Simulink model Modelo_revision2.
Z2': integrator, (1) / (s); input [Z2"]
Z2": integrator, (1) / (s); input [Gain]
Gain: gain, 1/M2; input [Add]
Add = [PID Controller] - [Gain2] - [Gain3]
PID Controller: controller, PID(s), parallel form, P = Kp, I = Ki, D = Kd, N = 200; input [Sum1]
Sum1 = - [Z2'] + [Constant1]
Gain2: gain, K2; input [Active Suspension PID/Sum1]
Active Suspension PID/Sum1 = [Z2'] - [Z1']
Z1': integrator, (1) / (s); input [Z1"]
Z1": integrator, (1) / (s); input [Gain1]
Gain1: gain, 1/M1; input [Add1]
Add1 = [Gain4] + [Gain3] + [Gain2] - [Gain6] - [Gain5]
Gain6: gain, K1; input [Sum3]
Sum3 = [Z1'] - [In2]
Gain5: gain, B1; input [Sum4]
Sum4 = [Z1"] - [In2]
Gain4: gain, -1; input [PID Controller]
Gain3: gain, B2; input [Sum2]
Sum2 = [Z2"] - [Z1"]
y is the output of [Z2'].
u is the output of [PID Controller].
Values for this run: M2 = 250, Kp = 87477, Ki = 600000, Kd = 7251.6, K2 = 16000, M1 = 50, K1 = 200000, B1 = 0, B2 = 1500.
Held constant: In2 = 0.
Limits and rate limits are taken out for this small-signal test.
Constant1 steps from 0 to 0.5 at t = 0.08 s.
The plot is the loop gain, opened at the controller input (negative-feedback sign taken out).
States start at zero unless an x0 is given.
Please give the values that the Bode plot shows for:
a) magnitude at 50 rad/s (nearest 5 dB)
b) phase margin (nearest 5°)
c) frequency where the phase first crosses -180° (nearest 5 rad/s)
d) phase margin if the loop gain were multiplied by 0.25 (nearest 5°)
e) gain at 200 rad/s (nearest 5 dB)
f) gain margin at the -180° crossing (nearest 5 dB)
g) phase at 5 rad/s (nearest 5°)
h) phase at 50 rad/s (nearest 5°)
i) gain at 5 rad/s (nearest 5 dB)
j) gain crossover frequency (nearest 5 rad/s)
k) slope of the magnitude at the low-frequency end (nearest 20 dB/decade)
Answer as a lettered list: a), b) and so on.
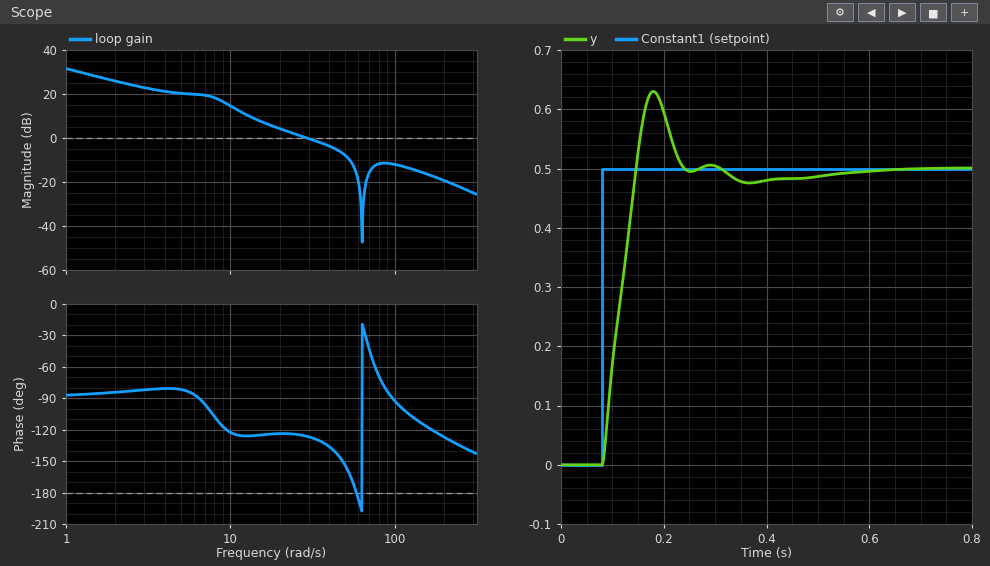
a) -10 dB
b) 55°
c) 60 rad/s
d) 55°
e) -20 dB
f) 15 dB
g) -80°
h) -155°
i) 20 dB
j) 30 rad/s
k) -20 dB/decade
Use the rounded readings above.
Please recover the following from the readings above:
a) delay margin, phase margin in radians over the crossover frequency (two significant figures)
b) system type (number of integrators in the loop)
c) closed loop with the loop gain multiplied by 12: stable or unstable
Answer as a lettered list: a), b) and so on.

a) 0.032 s
b) 1
c) unstable
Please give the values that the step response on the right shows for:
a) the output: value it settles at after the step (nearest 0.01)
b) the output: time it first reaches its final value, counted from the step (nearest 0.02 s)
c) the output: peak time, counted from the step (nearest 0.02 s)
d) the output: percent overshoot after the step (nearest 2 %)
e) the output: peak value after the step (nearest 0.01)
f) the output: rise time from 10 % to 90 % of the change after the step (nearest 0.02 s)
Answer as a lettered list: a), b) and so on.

a) 0.50
b) 0.06 s
c) 0.10 s
d) 26 %
e) 0.63
f) 0.06 s
